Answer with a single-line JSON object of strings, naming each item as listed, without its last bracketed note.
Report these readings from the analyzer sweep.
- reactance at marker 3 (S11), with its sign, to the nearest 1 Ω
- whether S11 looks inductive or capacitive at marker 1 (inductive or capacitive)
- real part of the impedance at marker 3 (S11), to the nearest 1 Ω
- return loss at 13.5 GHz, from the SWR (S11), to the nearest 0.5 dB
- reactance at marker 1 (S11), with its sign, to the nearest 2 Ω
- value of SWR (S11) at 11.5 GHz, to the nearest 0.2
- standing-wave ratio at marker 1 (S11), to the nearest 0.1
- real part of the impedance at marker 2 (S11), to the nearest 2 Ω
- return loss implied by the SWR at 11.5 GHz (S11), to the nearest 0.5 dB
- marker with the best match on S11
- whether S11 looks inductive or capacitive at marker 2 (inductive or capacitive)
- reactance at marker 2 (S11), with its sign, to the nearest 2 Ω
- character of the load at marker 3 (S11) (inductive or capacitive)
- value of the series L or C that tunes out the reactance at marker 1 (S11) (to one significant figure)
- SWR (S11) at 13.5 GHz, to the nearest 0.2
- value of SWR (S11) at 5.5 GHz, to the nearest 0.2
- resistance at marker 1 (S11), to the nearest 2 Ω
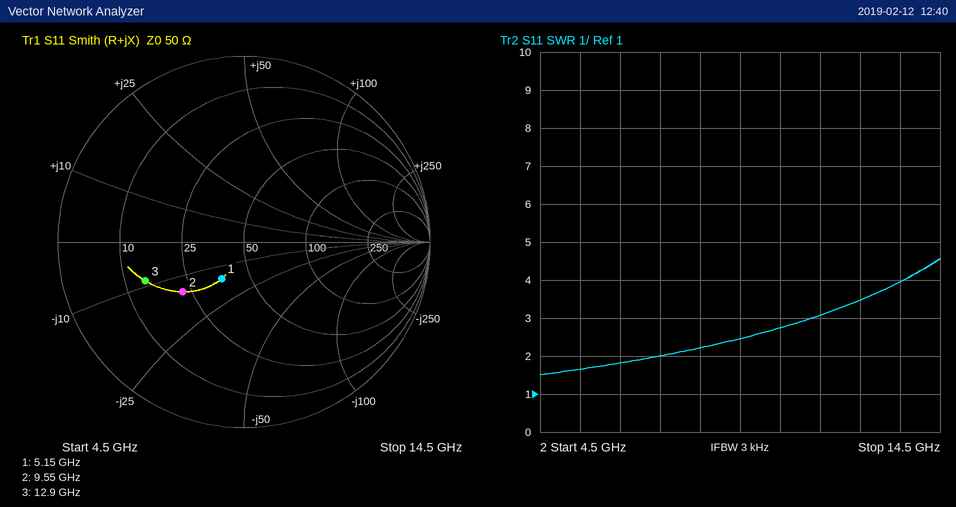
{"reactance at marker 3 (S11), with its sign, to the nearest 1 Ω": "-9 Ω", "whether S11 looks inductive or capacitive at marker 1": "capacitive", "real part of the impedance at marker 3 (S11), to the nearest 1 Ω": "14 Ω", "return loss at 13.5 GHz, from the SWR (S11), to the nearest 0.5 dB": "4.5 dB", "reactance at marker 1 (S11), with its sign, to the nearest 2 Ω": "-16 Ω", "value of SWR (S11) at 11.5 GHz, to the nearest 0.2": "3.0", "standing-wave ratio at marker 1 (S11), to the nearest 0.1": "1.6", "real part of the impedance at marker 2 (S11), to the nearest 2 Ω": "22 Ω", "return loss implied by the SWR at 11.5 GHz (S11), to the nearest 0.5 dB": "6.0 dB", "marker with the best match on S11": "marker 1", "whether S11 looks inductive or capacitive at marker 2": "capacitive", "reactance at marker 2 (S11), with its sign, to the nearest 2 Ω": "-14 Ω", "character of the load at marker 3 (S11)": "capacitive", "value of the series L or C that tunes out the reactance at marker 1 (S11)": "500 pH", "SWR (S11) at 13.5 GHz, to the nearest 0.2": "4.0", "value of SWR (S11) at 5.5 GHz, to the nearest 0.2": "1.6", "resistance at marker 1 (S11), to the nearest 2 Ω": "36 Ω"}
